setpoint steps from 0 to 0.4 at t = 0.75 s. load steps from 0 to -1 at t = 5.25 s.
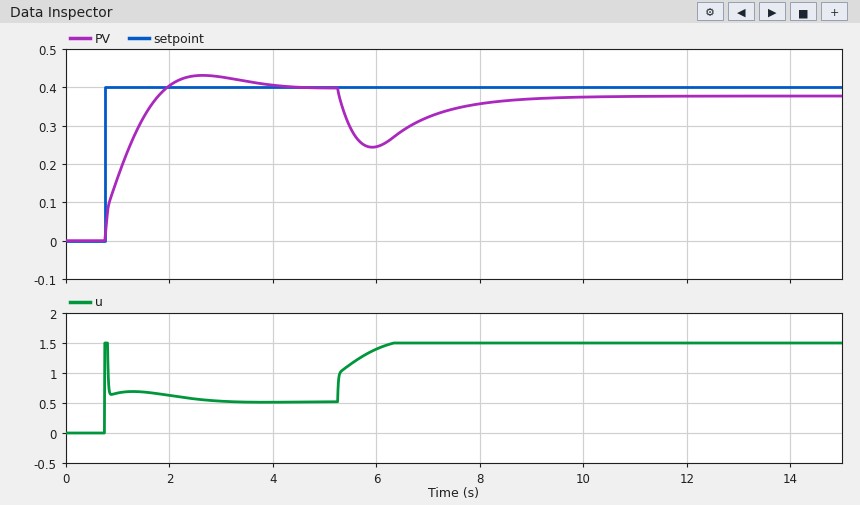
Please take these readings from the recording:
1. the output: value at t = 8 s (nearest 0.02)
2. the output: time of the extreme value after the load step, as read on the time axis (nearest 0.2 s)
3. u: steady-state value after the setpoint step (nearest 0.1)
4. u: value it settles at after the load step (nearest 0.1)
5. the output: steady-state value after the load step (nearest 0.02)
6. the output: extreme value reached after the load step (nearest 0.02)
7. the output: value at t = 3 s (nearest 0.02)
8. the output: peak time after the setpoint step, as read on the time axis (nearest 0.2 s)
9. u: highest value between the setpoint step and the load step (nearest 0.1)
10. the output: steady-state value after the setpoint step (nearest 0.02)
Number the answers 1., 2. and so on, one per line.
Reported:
1. 0.36
2. 6.0 s
3. 0.5
4. 1.5
5. 0.38
6. 0.24
7. 0.42
8. 2.6 s
9. 1.5
10. 0.40
